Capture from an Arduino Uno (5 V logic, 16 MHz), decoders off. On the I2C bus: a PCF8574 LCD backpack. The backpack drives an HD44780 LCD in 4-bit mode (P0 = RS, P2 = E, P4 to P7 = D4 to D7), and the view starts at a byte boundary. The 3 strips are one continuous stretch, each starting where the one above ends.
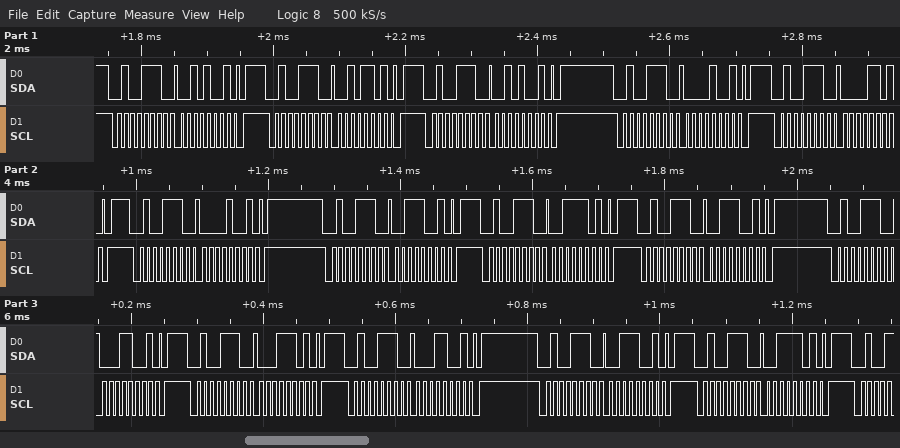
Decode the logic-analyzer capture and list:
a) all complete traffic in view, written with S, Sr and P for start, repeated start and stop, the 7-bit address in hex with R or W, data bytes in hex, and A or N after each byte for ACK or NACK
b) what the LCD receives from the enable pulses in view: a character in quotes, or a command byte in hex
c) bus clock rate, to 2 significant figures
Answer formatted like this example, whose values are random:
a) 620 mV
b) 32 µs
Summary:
a) S 27W A 29 A P S 27W A 2D A P S 27W A 29 A P S 27W A 09 A P S 27W A 0D A P S 27W A 09 A P S 27W A 39 A P S 27W A 3D A P S 27W A 39 A P S 27W A 19 A P S 27W A 1D A P S 27W A 19 A P S 27W A 39 A P S 27W A 3D A P
b) ' ' '1'
c) 100 kHz
